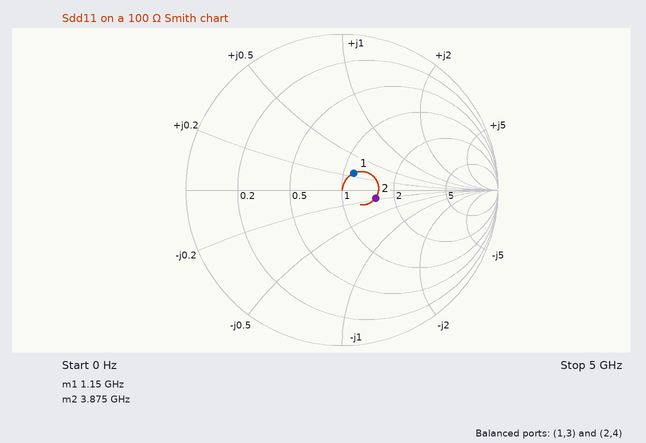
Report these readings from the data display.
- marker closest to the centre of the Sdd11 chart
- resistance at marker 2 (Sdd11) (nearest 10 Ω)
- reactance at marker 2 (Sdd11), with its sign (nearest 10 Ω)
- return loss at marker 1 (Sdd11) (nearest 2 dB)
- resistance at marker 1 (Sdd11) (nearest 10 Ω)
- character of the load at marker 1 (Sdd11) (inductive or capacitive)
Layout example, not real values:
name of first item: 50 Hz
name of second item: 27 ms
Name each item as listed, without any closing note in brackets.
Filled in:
marker closest to the centre of the Sdd11 chart: marker 1
resistance at marker 2 (Sdd11): 150 Ω
reactance at marker 2 (Sdd11), with its sign: -20 Ω
return loss at marker 1 (Sdd11): 18 dB
resistance at marker 1 (Sdd11): 110 Ω
character of the load at marker 1 (Sdd11): inductive
